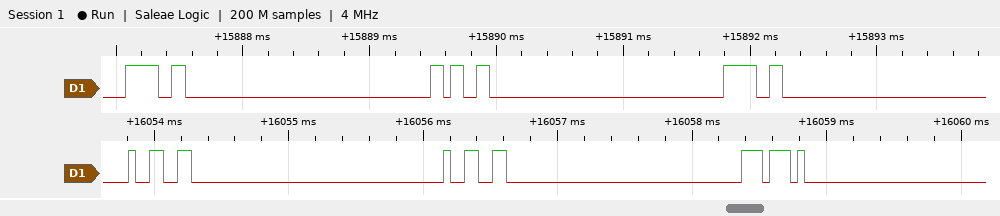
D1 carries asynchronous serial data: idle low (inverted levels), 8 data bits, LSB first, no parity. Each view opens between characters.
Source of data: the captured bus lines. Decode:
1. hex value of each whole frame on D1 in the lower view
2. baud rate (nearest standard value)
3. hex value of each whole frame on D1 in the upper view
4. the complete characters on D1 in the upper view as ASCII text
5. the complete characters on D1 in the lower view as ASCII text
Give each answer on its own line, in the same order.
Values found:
33, 33, 44
19200 baud
30, 32, 30
"020"
"33D"
